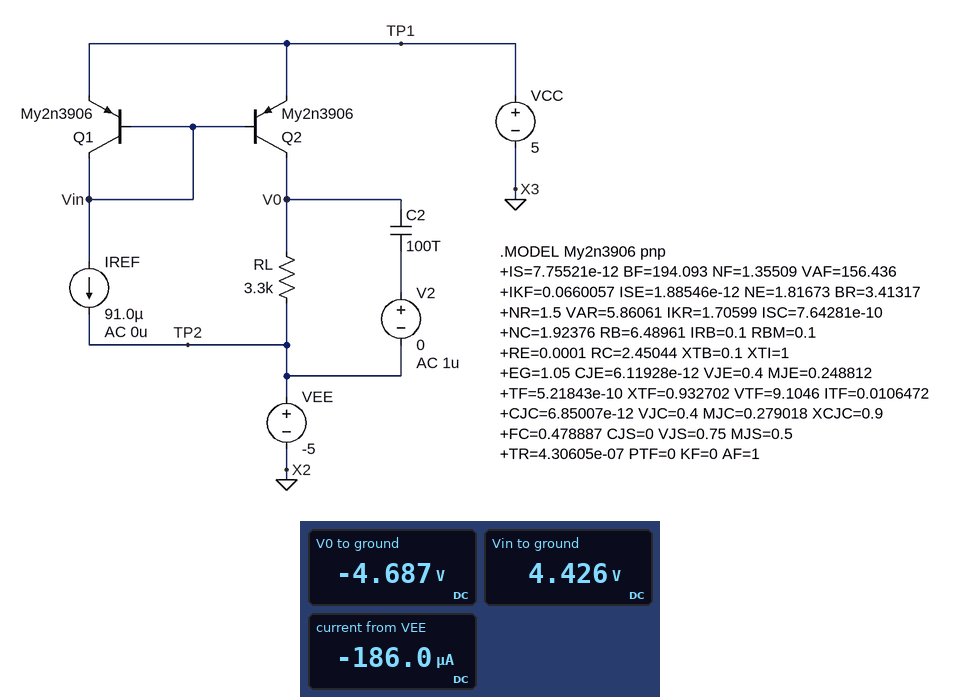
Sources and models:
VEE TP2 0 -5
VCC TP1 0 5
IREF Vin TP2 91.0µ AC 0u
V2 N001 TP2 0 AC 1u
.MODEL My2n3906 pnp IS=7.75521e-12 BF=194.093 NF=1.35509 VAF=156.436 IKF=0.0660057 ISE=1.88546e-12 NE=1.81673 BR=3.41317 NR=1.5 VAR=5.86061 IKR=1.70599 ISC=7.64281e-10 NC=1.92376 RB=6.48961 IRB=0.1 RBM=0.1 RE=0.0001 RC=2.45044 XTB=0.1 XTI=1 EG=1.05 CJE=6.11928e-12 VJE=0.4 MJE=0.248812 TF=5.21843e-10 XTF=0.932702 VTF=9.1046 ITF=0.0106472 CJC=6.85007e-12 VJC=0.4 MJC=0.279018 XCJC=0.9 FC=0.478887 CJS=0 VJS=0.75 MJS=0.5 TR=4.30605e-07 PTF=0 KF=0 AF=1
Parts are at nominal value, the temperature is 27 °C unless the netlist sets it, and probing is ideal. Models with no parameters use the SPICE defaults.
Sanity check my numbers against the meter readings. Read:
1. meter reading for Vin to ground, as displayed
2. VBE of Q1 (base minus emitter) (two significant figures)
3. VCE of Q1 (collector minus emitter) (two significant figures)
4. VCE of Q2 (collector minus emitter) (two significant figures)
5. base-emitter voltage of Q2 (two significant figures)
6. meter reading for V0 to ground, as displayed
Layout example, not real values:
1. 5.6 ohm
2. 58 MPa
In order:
1. 4.426 V
2. -570 mV
3. -570 mV
4. -9.7 V
5. -570 mV
6. -4.687 V
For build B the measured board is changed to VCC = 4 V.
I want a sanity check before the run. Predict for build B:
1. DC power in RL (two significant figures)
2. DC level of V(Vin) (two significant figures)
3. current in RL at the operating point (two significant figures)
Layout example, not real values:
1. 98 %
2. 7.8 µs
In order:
1. 29 µW
2. 3.4 V
3. 94 µA
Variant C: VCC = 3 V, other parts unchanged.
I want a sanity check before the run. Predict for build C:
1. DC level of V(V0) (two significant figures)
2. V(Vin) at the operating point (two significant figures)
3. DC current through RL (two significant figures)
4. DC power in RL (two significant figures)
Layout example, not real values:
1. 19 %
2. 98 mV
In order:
1. -4.7 V
2. 2.4 V
3. 94 µA
4. 29 µW
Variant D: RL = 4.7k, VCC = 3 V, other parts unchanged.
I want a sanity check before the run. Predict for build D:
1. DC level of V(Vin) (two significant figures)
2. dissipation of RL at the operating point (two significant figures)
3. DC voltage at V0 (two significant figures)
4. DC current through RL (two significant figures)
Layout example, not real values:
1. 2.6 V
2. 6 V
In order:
1. 2.4 V
2. 41 µW
3. -4.6 V
4. 94 µA
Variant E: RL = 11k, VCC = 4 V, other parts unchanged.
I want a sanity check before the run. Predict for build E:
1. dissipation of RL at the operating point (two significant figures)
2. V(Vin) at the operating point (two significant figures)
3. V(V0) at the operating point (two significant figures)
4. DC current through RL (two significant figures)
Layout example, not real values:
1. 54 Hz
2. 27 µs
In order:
1. 97 µW
2. 3.4 V
3. -4.0 V
4. 94 µA
